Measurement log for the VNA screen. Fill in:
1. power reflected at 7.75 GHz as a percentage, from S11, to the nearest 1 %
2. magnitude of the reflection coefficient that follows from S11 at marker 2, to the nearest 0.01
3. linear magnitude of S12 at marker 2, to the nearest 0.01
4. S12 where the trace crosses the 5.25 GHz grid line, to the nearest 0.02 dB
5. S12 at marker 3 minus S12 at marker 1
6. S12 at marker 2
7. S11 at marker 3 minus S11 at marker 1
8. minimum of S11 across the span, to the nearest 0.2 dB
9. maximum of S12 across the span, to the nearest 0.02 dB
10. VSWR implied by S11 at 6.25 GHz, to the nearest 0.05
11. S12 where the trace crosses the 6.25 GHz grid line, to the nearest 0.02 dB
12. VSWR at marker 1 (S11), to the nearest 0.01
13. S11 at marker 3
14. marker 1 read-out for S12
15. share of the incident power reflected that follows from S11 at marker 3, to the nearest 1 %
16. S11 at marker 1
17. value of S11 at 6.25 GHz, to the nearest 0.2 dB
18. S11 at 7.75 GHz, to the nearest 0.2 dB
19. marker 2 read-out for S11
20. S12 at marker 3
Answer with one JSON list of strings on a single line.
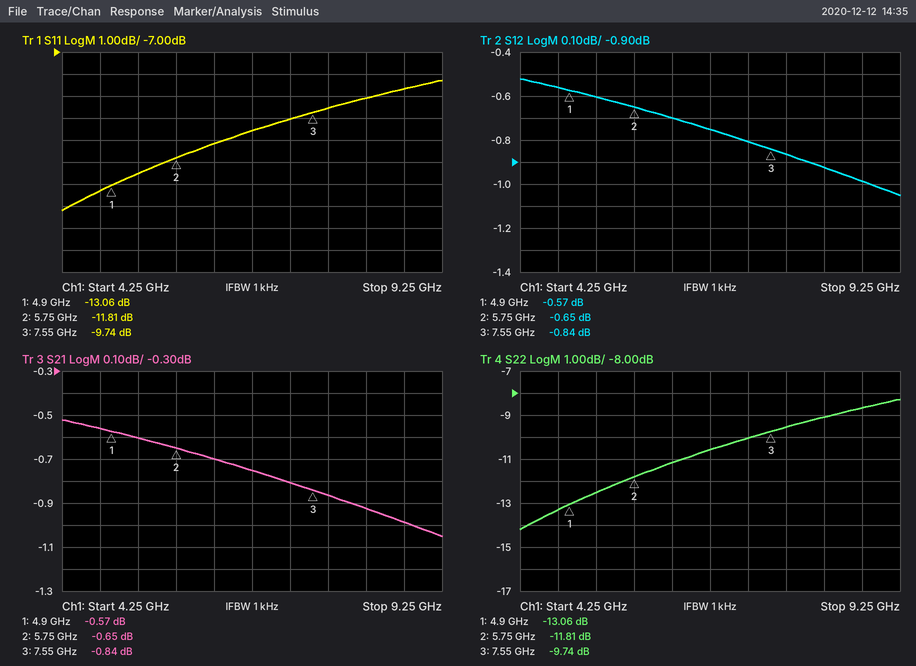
["11 %", "0.26", "0.93", "-0.60 dB", "-0.27 dB", "-0.65 dB", "3.32 dB", "-14.2 dB", "-0.52 dB", "1.75", "-0.70 dB", "1.57", "-9.74 dB", "-0.57 dB", "11 %", "-13.06 dB", "-11.2 dB", "-9.6 dB", "-11.81 dB", "-0.84 dB"]
